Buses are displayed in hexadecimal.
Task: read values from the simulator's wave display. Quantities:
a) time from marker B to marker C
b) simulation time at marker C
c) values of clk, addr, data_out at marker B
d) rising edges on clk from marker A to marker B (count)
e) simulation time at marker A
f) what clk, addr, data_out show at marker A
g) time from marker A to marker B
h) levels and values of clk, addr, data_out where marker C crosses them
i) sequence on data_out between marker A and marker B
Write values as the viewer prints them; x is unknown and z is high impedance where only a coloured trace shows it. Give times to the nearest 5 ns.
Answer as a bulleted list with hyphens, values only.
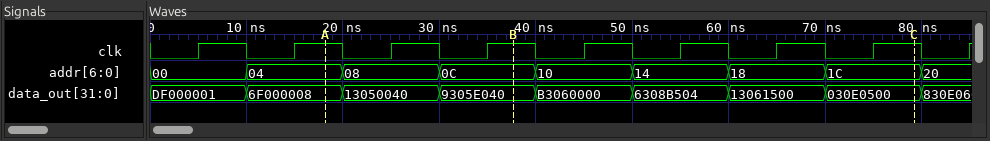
- 40 ns
- 80 ns
- clk=1, addr=0C, data_out=9305E040
- 2
- 20 ns
- clk=1, addr=04, data_out=6F000008
- 20 ns
- clk=1, addr=1C, data_out=030E0500
- 6F000008, 13050040, 9305E040
